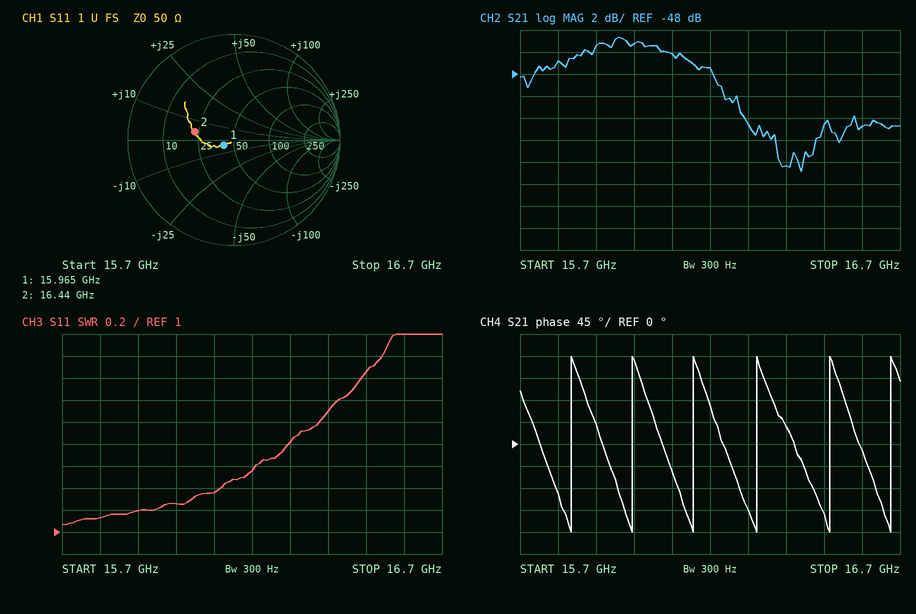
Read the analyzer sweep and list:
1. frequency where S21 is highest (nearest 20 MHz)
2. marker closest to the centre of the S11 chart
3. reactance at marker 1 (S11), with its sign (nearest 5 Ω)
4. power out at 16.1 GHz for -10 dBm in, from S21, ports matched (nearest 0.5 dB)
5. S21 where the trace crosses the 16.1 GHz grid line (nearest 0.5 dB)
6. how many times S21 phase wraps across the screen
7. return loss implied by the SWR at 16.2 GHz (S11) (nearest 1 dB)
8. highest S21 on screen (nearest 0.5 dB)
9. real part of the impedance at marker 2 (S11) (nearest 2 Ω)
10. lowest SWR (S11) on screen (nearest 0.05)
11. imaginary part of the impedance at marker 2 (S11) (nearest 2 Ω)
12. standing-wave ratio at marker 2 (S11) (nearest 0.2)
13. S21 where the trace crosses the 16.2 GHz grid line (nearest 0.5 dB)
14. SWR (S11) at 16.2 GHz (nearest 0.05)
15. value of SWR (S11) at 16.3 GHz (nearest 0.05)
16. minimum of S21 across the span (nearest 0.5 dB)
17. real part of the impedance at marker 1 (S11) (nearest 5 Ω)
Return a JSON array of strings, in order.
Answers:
["15.96 GHz", "marker 1", "-5 Ω", "-56.0 dBm", "-46.0 dB", "6", "13 dB", "-44.5 dB", "22 Ω", "1.05", "+4 Ω", "2.2", "-47.5 dB", "1.55", "1.80", "-57.0 dB", "40 Ω"]
